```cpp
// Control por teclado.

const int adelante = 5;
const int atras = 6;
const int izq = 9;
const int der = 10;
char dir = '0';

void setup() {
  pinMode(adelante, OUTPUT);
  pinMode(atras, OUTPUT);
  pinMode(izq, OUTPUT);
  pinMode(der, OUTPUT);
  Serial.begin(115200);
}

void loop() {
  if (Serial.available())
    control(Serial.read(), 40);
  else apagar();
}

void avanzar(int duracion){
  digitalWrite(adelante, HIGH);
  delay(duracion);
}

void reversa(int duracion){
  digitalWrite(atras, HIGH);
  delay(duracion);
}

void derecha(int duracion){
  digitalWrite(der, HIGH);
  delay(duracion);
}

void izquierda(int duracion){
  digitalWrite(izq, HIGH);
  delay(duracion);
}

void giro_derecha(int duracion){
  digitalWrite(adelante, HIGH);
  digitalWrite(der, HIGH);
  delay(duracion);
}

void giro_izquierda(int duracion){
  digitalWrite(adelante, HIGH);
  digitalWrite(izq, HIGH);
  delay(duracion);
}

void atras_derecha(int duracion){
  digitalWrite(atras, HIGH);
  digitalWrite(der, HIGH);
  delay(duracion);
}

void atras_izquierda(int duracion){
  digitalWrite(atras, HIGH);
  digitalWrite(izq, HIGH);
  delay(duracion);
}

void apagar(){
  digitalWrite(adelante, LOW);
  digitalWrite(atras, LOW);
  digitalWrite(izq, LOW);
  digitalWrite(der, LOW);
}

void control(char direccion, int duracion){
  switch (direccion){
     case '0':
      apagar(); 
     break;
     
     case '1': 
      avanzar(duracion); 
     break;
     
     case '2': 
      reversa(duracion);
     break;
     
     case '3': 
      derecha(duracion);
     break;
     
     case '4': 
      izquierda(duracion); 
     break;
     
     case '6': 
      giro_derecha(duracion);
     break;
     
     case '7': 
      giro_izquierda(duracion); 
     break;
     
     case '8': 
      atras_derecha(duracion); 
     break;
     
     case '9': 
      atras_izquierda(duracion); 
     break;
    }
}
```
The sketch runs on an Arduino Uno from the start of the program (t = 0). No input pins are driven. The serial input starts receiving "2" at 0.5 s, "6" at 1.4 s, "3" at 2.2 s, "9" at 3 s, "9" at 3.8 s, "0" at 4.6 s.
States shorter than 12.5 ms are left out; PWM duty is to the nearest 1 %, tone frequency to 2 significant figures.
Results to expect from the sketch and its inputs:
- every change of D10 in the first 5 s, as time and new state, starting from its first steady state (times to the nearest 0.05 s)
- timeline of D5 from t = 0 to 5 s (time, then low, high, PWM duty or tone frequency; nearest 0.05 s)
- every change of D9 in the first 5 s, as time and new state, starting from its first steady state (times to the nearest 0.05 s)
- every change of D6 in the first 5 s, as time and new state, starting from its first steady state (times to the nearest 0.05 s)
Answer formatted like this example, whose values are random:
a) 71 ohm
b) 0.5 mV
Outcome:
a) 0 s low; 1.4 s high; 1.45 s low; 2.2 s high; 2.25 s low
b) 0 s low; 1.4 s high; 1.45 s low
c) 0 s low; 3 s high; 3.05 s low; 3.8 s high; 3.85 s low
d) 0 s low; 0.5 s high; 0.55 s low; 3 s high; 3.05 s low; 3.8 s high; 3.85 s low
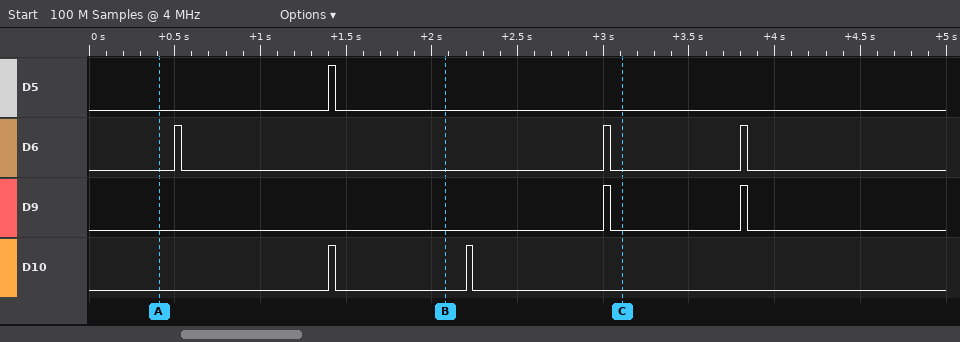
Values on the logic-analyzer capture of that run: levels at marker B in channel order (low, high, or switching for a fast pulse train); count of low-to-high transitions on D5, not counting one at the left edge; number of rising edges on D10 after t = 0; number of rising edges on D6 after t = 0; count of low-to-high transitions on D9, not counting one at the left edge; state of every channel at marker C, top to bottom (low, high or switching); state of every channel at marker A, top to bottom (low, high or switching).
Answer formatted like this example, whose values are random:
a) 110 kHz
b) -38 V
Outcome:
a) D5 low, D6 low, D9 low, D10 low
b) 1
c) 2
d) 3
e) 2
f) D5 low, D6 low, D9 low, D10 low
g) D5 low, D6 low, D9 low, D10 low
